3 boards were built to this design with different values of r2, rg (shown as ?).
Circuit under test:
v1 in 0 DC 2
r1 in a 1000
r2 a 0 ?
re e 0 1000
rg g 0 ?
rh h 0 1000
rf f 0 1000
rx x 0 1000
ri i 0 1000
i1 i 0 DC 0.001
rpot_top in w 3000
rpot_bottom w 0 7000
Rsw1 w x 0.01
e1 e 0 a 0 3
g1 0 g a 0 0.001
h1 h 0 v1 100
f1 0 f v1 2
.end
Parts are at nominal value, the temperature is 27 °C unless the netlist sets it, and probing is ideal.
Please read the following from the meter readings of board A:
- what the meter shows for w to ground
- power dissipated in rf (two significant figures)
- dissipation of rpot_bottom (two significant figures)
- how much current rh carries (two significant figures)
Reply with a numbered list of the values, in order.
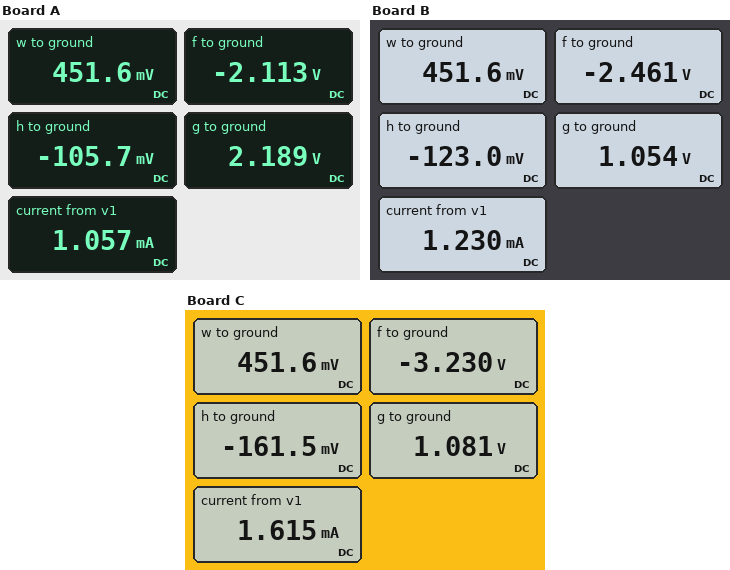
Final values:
1. 451.6 mV
2. 4.5 mW
3. 29 µW
4. 110 µA
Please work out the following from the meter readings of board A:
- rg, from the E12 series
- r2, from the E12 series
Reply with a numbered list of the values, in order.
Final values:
1. 1.5 kΩ
2. 2.7 kΩ
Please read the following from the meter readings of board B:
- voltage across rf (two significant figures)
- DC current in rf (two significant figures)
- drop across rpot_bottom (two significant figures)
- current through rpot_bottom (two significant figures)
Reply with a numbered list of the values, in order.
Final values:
1. 2.5 V
2. 2.5 mA
3. 450 mV
4. 65 µA
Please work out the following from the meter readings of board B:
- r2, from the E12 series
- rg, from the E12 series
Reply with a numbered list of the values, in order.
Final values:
1. 1.8 kΩ
2. 820 Ω
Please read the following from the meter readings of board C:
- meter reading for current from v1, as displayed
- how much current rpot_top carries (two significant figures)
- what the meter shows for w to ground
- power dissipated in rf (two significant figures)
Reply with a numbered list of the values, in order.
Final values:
1. 1.615 mA
2. 520 µA
3. 451.6 mV
4. 10 mW
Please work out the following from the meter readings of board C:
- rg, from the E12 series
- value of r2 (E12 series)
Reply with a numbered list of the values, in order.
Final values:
1. 1.2 kΩ
2. 820 Ω
